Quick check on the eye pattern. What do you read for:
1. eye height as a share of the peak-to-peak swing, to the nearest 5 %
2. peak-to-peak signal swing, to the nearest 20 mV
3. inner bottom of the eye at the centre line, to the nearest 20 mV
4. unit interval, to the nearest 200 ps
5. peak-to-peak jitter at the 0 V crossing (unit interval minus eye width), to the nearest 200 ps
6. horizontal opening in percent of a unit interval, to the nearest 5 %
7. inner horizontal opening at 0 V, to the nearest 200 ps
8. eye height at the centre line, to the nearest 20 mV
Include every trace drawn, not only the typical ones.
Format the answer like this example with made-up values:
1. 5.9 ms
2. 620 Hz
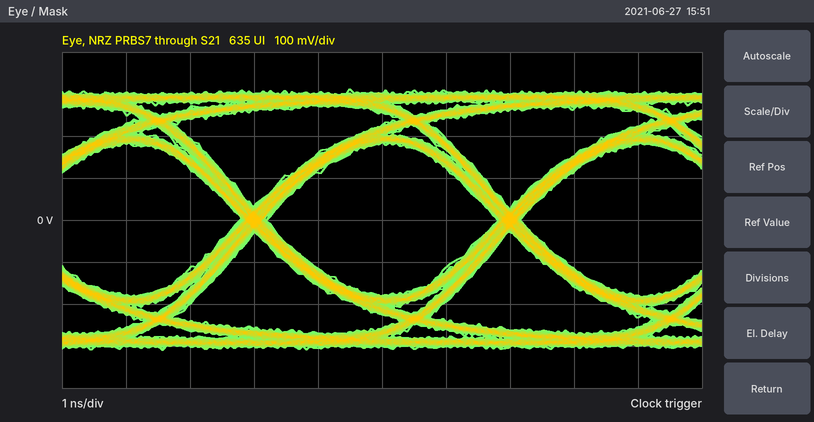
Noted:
1. 60 %
2. 620 mV
3. -180 mV
4. 4.0 ns
5. 400 ps
6. 90 %
7. 3.6 ns
8. 360 mV
